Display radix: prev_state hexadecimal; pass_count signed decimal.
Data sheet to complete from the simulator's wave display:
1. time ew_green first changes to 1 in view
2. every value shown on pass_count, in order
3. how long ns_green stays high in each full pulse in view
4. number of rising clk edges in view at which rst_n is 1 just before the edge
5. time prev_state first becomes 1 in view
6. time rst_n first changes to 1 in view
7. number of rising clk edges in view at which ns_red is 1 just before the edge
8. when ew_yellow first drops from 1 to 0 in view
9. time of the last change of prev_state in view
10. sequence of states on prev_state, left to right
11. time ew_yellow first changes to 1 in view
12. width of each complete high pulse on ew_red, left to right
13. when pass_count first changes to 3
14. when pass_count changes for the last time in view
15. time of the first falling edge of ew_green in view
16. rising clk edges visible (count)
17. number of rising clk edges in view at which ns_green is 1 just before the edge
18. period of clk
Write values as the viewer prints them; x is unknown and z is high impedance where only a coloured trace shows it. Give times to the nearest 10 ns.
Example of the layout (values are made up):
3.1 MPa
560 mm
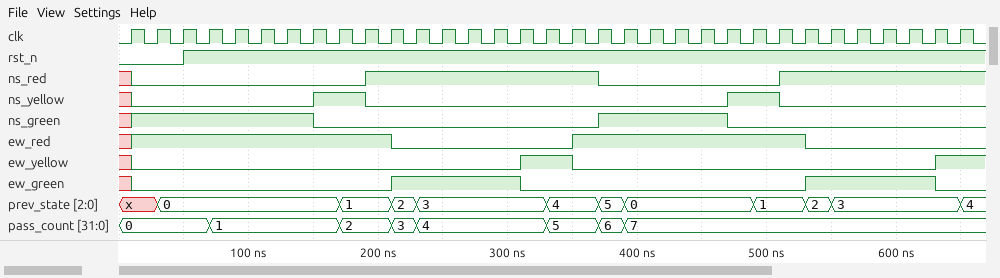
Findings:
210 ns
0, 1, 2, 3, 4, 5, 6, 7
100 ns
30
170 ns
50 ns
16
350 ns
650 ns
x, 0, 1, 2, 3, 4, 5, 0, 1, 2, 3, 4
310 ns
180 ns
210 ns
390 ns
310 ns
33
12
20 ns
